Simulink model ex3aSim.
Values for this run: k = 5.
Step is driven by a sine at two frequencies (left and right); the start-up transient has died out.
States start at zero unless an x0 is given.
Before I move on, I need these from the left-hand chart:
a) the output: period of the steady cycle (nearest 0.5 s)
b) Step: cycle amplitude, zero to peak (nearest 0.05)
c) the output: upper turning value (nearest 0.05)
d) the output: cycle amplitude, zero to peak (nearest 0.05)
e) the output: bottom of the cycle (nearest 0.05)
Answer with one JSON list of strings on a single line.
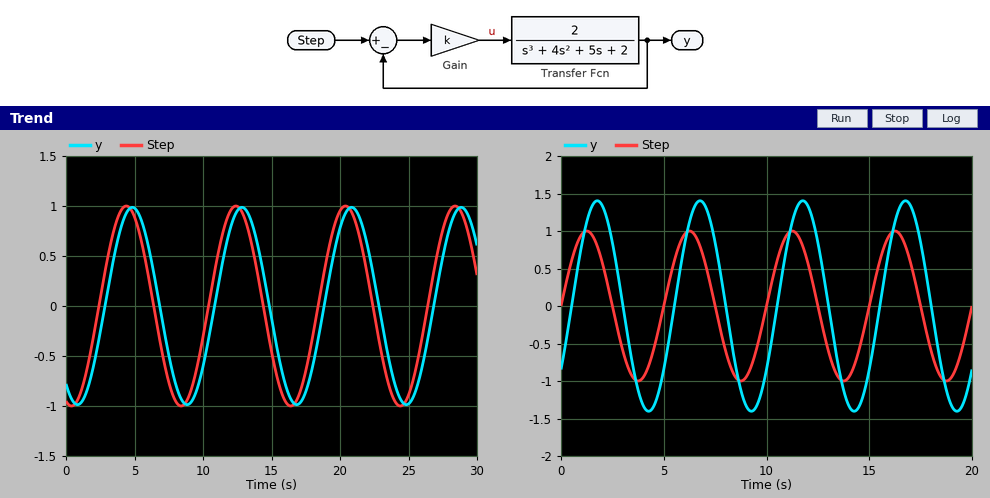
["8.0 s", "1.00", "1.00", "1.00", "-1.00"]
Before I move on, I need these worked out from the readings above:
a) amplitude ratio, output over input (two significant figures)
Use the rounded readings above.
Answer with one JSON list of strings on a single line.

["1.0"]
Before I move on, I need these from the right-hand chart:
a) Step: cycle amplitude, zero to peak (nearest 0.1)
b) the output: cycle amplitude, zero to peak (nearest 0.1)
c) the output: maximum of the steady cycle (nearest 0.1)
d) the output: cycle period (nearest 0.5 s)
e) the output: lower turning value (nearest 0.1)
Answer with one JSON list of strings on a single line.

["1.0", "1.4", "1.4", "5.0 s", "-1.4"]
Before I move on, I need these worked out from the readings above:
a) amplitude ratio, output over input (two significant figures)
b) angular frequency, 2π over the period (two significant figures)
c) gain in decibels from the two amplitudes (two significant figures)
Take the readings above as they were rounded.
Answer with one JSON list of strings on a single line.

["1.4", "1.3 rad/s", "2.9 dB"]
